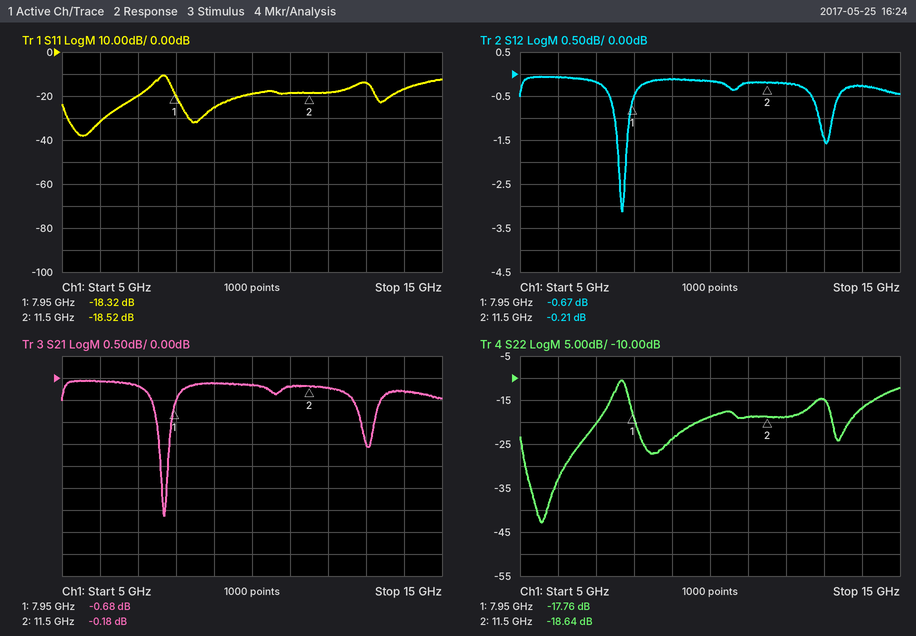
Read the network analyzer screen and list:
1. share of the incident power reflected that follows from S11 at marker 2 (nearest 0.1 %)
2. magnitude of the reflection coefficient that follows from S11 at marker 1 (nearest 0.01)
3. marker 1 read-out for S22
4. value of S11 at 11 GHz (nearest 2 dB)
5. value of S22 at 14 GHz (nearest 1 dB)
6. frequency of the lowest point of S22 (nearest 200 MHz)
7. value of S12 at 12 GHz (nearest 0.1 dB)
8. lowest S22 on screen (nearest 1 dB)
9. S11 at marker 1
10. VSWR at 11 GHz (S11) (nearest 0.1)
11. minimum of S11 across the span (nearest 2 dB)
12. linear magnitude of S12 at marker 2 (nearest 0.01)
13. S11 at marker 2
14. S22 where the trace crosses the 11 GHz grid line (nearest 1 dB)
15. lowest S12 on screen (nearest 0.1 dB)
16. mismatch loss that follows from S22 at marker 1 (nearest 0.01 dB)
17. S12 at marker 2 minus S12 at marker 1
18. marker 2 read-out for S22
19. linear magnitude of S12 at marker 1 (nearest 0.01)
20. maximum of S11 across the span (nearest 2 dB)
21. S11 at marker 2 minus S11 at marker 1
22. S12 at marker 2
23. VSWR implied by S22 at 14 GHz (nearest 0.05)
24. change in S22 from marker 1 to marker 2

1.4 %
0.12
-17.76 dB
-18 dB
-17 dB
5.6 GHz
-0.2 dB
-43 dB
-18.32 dB
1.3
-38 dB
0.98
-18.52 dB
-19 dB
-3.1 dB
0.07 dB
0.46 dB
-18.64 dB
0.93
-10 dB
-0.20 dB
-0.21 dB
1.35
-0.88 dB
